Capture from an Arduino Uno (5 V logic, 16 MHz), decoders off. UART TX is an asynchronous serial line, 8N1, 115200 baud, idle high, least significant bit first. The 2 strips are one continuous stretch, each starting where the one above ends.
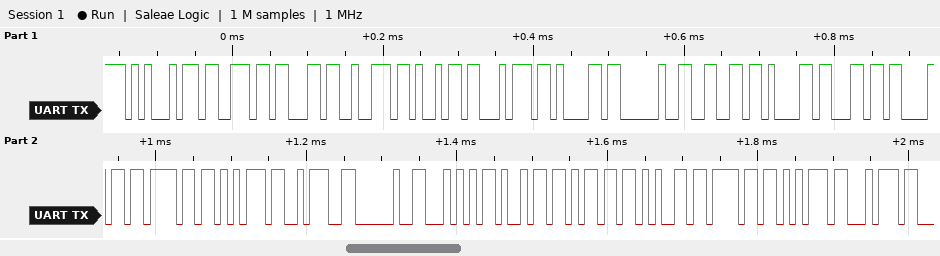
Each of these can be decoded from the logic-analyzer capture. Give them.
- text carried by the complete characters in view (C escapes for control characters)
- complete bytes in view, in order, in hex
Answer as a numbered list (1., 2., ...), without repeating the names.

1. "Escrita falhou: Timeout"
2. 0x45 0x73 0x63 0x72 0x69 0x74 0x61 0x20 0x66 0x61 0x6C 0x68 0x6F 0x75 0x3A 0x20 0x54 0x69 0x6D 0x65 0x6F 0x75 0x74
